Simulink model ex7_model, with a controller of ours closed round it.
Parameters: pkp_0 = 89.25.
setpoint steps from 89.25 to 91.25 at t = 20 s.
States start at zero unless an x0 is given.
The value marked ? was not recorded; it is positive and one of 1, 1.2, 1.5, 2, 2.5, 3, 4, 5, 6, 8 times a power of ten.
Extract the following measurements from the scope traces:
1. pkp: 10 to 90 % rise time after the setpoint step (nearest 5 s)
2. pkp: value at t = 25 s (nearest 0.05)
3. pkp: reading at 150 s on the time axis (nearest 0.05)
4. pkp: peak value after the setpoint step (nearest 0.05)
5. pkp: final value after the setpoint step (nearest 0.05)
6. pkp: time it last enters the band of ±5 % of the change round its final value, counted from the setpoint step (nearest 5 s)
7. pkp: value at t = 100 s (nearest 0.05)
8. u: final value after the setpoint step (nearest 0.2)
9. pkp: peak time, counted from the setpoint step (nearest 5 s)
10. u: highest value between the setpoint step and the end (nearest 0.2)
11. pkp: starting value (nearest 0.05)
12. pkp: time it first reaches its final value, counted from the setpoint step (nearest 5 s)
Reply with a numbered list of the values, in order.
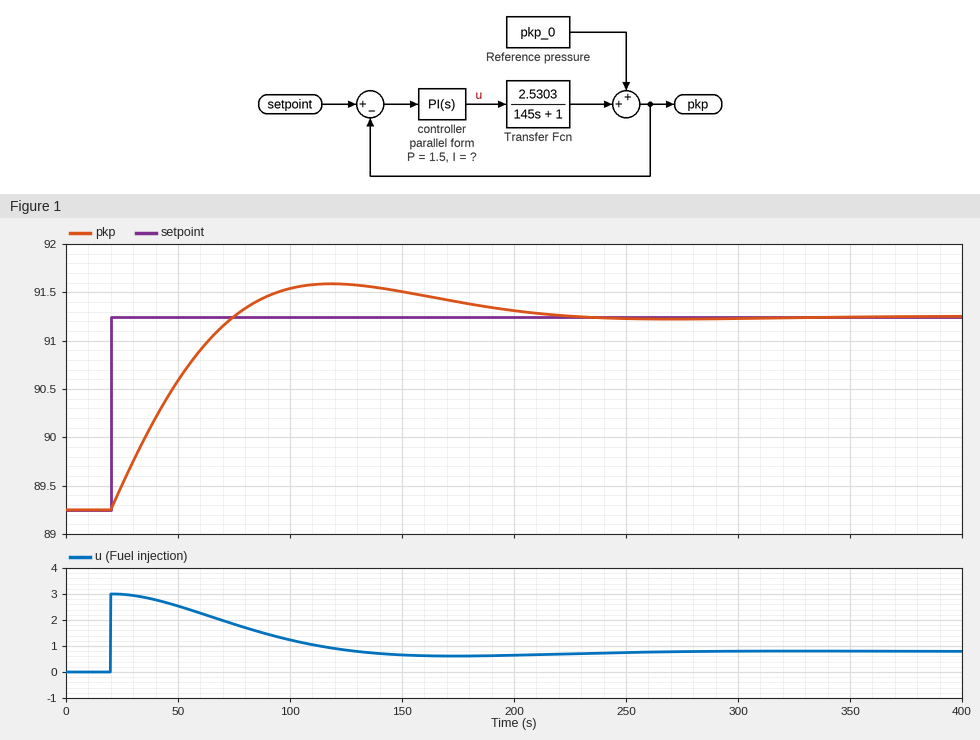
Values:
1. 40 s
2. 89.50
3. 91.50
4. 91.60
5. 91.25
6. 170 s
7. 91.55
8. 0.8
9. 100 s
10. 3.0
11. 89.25
12. 55 s
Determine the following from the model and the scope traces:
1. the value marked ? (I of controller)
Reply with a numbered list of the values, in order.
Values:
1. 0.04
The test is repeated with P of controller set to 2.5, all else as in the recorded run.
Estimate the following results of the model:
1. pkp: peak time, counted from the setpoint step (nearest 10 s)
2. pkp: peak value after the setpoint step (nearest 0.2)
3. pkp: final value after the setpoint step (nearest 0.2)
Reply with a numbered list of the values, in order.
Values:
1. 90 s
2. 91.4
3. 91.2
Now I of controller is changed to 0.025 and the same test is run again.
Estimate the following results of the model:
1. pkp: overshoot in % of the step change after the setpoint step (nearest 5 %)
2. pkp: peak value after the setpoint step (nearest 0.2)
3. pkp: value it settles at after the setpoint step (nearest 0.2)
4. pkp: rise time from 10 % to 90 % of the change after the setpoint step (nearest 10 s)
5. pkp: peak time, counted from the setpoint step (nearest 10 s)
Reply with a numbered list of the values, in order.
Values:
1. 10 %
2. 91.4
3. 91.2
4. 50 s
5. 120 s
